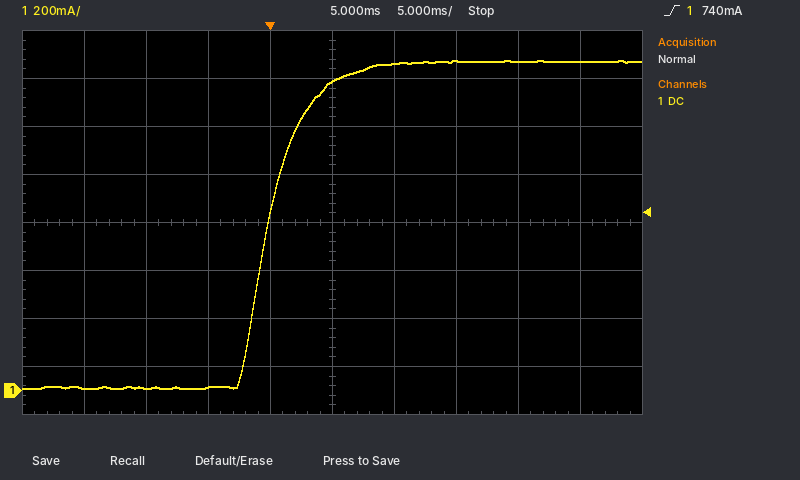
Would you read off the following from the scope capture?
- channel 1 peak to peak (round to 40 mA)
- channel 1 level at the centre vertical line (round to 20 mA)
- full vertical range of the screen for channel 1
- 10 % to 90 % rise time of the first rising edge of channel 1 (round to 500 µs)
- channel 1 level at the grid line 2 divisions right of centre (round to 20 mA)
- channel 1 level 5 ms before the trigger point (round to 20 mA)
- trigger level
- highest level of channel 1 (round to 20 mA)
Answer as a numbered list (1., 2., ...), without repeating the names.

1. 1.36 A
2. 1.28 A
3. 1.6 A
4. 6.0 ms
5. 1.38 A
6. 20 mA
7. 740 mA
8. 1.38 A
